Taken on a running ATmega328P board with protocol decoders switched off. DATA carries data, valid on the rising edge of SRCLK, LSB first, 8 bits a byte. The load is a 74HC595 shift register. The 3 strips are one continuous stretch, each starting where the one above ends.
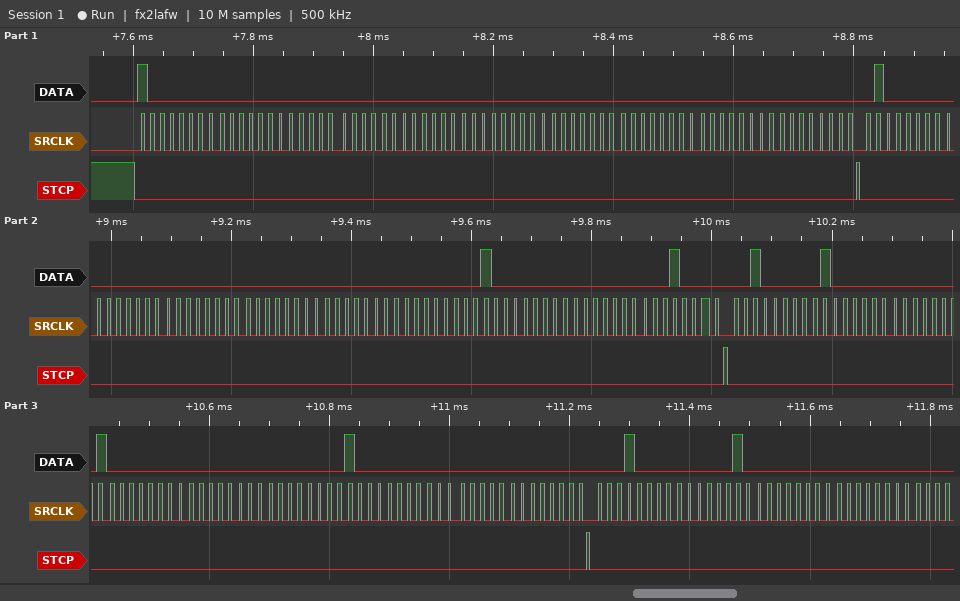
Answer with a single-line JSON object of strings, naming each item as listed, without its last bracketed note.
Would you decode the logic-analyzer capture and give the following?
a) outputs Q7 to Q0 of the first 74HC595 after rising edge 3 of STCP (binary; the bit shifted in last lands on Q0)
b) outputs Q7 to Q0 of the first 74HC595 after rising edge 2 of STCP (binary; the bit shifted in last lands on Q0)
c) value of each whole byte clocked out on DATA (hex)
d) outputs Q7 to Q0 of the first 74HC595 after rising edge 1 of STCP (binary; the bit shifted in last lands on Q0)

{"outputs Q7 to Q0 of the first 74HC595 after rising edge 3 of STCP": "00000000", "outputs Q7 to Q0 of the first 74HC595 after rising edge 2 of STCP": "00010000", "value of each whole byte clocked out on DATA": "01 00 00 00 00 00 00 00 00 02 00 00 00 00 00 01 00 08 04 02 80 00 00 00 01 00 00 08 40 00 00", "outputs Q7 to Q0 of the first 74HC595 after rising edge 1 of STCP": "00000000"}
